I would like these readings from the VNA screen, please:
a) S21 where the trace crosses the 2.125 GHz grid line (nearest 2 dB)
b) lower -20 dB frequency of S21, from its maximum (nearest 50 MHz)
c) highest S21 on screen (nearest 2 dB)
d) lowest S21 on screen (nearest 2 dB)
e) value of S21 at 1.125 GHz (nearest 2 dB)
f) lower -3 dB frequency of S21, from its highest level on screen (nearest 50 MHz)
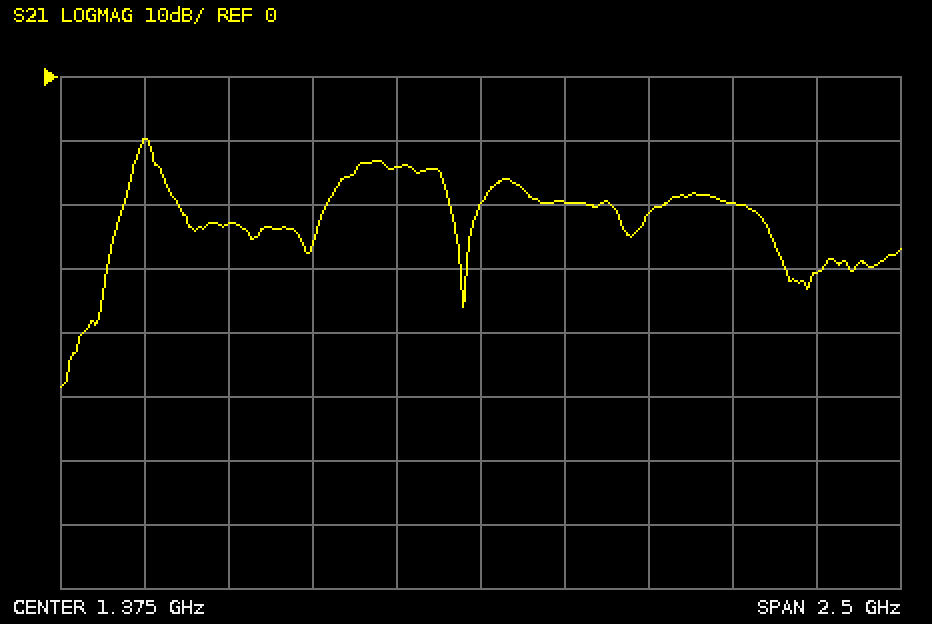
-20 dB
250 MHz
-10 dB
-48 dB
-14 dB
350 MHz
